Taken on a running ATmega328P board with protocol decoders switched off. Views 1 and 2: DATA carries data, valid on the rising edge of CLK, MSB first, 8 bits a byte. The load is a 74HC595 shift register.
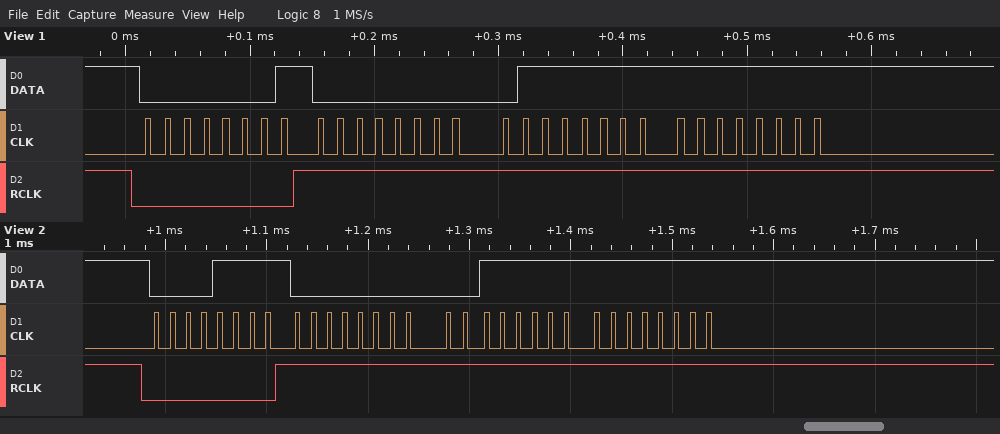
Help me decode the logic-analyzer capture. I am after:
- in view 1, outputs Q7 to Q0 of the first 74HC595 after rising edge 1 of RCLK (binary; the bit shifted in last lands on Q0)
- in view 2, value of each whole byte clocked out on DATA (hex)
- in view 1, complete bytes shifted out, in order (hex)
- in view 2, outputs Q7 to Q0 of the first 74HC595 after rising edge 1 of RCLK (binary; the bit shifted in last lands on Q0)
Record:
00000001
0x0F 0x00 0x3F 0xFF
01 00 7F FF
00001111
